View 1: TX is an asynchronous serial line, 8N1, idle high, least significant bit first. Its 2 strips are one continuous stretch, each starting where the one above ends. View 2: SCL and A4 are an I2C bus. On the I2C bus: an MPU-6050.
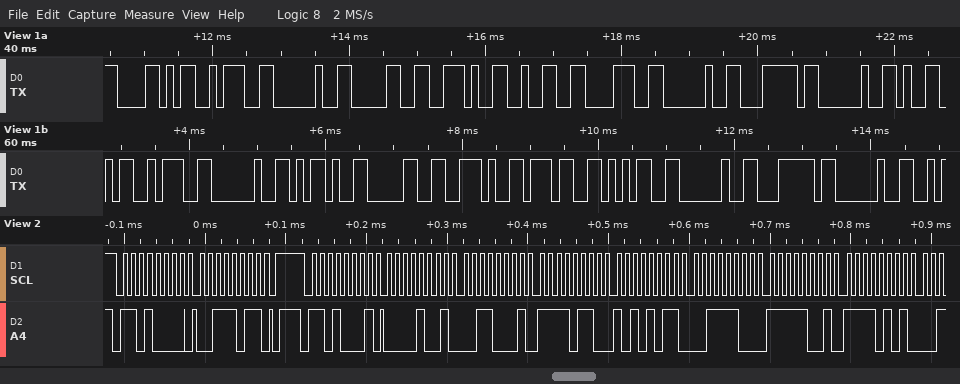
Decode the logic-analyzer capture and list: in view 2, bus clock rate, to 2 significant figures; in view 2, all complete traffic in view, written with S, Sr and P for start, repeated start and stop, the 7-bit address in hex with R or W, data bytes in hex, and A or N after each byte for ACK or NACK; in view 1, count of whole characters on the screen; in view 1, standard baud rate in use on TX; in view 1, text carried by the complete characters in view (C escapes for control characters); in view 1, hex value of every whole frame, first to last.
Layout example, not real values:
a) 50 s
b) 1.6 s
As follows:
a) 100 kHz
b) S 68W A 3B A P S 68R A 09 A 31 A F6 A AB A 3C A F9 A F5 A
c) 21
d) 9600 baud
e) "X: 0.28 | Y: -0.75 | "
f) 58 3A 20 30 2E 32 38 20 7C 20 59 3A 20 2D 30 2E 37 35 20 7C 20
